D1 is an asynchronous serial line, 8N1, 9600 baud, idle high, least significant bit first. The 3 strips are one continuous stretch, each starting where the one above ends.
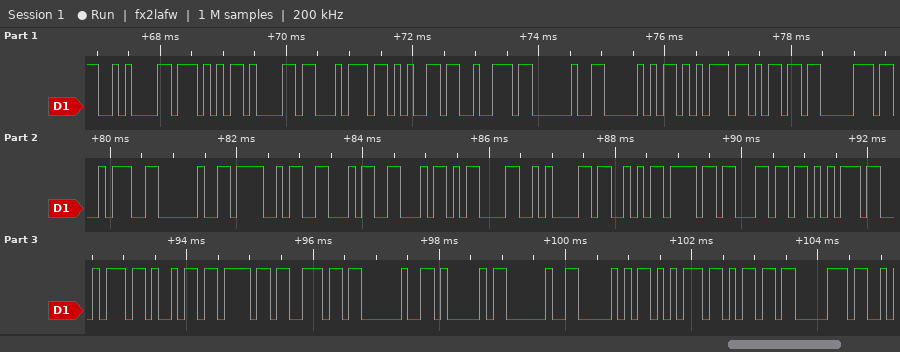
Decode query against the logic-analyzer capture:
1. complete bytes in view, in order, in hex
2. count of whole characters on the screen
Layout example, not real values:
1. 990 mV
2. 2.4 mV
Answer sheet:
1. 0A 57 61 74 65 72 20 50 75 6D 70 3A 20 4F 46 46 0D 0A 53 6F 6C 75 74 69 6F 6E 20 41 20 50 75 6D 70
2. 33
